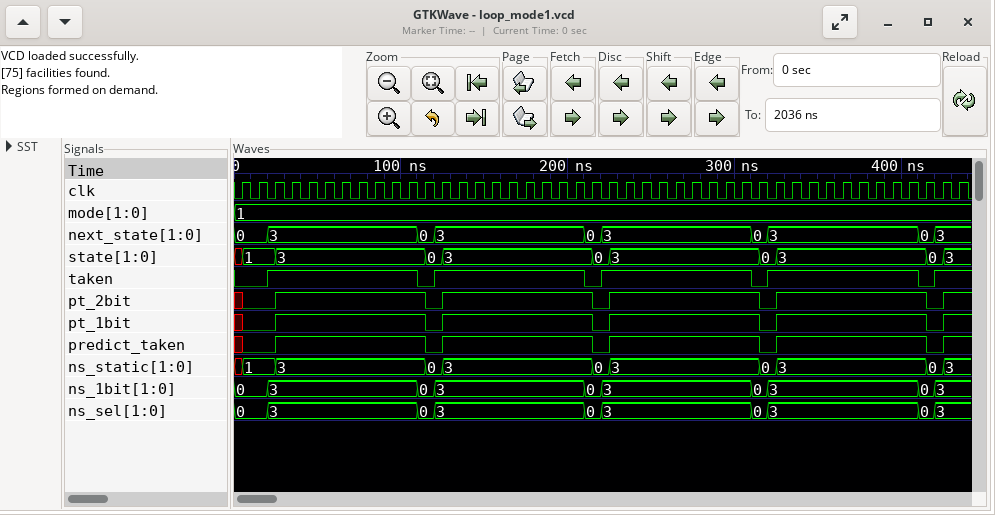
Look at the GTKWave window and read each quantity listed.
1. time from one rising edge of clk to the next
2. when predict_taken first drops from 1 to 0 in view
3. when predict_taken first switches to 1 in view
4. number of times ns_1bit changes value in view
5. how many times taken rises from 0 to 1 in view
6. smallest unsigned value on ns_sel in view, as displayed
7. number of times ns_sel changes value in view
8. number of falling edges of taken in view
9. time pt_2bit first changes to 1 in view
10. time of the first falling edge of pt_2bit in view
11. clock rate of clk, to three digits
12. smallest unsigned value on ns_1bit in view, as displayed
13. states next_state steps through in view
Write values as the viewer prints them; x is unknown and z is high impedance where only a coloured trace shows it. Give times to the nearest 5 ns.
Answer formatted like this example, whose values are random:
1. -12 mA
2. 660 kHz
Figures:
1. 10 ns
2. 115 ns
3. 25 ns
4. 9
5. 5
6. 0
7. 9
8. 4
9. 25 ns
10. 115 ns
11. 100 MHz
12. 0
13. 0, 3, 0, 3, 0, 3, 0, 3, 0, 3
